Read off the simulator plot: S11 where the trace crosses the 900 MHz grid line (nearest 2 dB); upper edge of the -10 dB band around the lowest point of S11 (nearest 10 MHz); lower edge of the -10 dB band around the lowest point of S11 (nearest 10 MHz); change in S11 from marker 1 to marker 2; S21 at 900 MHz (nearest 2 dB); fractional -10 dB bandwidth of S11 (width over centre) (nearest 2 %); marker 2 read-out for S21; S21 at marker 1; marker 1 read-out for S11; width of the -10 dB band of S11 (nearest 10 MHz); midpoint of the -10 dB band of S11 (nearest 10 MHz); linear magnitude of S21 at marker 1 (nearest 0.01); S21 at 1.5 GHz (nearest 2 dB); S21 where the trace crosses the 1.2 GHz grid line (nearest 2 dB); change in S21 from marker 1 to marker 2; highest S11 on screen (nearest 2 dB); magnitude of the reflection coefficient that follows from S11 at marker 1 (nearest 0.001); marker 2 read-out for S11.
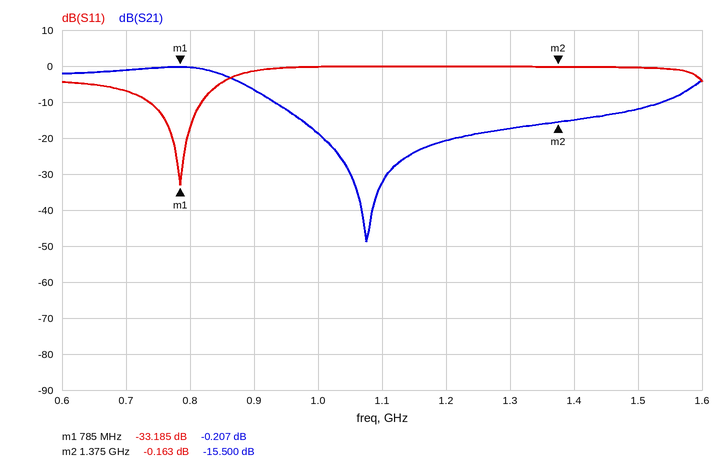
-2 dB
820 MHz
740 MHz
33.022 dB
-6 dB
10 %
-15.500 dB
-0.207 dB
-33.185 dB
80 MHz
780 MHz
0.98
-12 dB
-20 dB
-15.293 dB
0 dB
0.022
-0.163 dB
